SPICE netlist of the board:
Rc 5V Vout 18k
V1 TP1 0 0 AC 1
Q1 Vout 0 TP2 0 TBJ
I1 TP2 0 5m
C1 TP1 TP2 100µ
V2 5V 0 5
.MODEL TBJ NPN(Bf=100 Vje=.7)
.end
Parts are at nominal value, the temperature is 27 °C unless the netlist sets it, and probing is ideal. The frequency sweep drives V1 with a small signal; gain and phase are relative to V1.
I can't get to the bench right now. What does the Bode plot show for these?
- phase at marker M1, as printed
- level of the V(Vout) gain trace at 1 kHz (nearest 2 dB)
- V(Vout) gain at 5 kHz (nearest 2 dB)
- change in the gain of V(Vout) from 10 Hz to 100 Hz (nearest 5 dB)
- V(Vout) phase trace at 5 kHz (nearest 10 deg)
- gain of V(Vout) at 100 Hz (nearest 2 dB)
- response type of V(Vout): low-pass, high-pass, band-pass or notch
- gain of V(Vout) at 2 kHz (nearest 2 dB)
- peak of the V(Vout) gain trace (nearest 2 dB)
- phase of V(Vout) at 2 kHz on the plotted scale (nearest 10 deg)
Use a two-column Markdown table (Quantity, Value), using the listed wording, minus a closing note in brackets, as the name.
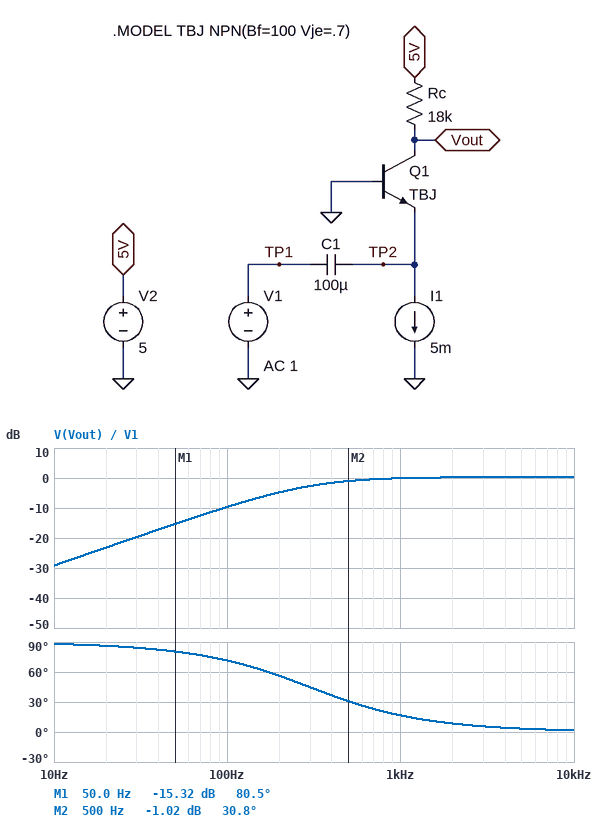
| Quantity | Value |
|---|---|
| phase at marker M1, as printed | 80.5 deg |
| level of the V(Vout) gain trace at 1 kHz | 0 dB |
| V(Vout) gain at 5 kHz | 0 dB |
| change in the gain of V(Vout) from 10 Hz to 100 Hz | 20 dB |
| V(Vout) phase trace at 5 kHz | 0 deg |
| gain of V(Vout) at 100 Hz | -10 dB |
| response type of V(Vout): low-pass, high-pass, band-pass or notch | high-pass |
| gain of V(Vout) at 2 kHz | 0 dB |
| peak of the V(Vout) gain trace | 0 dB |
| phase of V(Vout) at 2 kHz on the plotted scale | 10 deg |
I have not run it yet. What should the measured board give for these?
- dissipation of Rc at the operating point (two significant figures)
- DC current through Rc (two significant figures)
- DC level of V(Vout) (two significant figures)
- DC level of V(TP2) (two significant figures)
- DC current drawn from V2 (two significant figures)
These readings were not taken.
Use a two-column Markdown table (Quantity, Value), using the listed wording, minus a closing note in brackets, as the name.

| Quantity | Value |
|---|---|
| dissipation of Rc at the operating point | 1.9 mW |
| DC current through Rc | 320 µA |
| DC level of V(Vout) | -810 mV |
| DC level of V(TP2) | -830 mV |
| DC current drawn from V2 | 320 µA |
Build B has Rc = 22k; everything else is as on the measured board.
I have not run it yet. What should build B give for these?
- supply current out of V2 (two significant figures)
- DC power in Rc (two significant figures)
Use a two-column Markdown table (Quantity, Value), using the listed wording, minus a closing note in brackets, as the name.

| Quantity | Value |
|---|---|
| supply current out of V2 | 260 µA |
| DC power in Rc | 1.5 mW |
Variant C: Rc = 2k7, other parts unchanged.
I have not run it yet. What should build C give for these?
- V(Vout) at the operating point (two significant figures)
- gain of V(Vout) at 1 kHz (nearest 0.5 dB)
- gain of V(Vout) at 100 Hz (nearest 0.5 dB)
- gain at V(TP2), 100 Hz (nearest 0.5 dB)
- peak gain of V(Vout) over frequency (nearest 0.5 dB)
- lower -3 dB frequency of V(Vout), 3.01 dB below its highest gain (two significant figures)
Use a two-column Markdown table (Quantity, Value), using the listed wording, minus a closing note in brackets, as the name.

| Quantity | Value |
|---|---|
| V(Vout) at the operating point | -800 mV |
| gain of V(Vout) at 1 kHz | 2.5 dB |
| gain of V(Vout) at 100 Hz | -5.5 dB |
| gain at V(TP2), 100 Hz | -8.5 dB |
| peak gain of V(Vout) over frequency | 3.0 dB |
| lower -3 dB frequency of V(Vout), 3.01 dB below its highest gain | 240 Hz |
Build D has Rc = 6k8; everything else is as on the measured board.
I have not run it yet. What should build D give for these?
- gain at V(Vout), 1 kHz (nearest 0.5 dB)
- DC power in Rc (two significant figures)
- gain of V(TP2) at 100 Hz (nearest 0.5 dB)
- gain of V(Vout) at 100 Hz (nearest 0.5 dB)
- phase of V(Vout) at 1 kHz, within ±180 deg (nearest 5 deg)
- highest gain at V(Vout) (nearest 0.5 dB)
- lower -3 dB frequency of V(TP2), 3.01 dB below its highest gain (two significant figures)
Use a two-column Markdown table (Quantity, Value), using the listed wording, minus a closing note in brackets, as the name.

| Quantity | Value |
|---|---|
| gain at V(Vout), 1 kHz | 0.5 dB |
| DC power in Rc | 5.0 mW |
| gain of V(TP2) at 100 Hz | -9.5 dB |
| gain of V(Vout) at 100 Hz | -8.5 dB |
| phase of V(Vout) at 1 kHz, within ±180 deg | 15 deg |
| highest gain at V(Vout) | 1.0 dB |
| lower -3 dB frequency of V(TP2), 3.01 dB below its highest gain | 280 Hz |
